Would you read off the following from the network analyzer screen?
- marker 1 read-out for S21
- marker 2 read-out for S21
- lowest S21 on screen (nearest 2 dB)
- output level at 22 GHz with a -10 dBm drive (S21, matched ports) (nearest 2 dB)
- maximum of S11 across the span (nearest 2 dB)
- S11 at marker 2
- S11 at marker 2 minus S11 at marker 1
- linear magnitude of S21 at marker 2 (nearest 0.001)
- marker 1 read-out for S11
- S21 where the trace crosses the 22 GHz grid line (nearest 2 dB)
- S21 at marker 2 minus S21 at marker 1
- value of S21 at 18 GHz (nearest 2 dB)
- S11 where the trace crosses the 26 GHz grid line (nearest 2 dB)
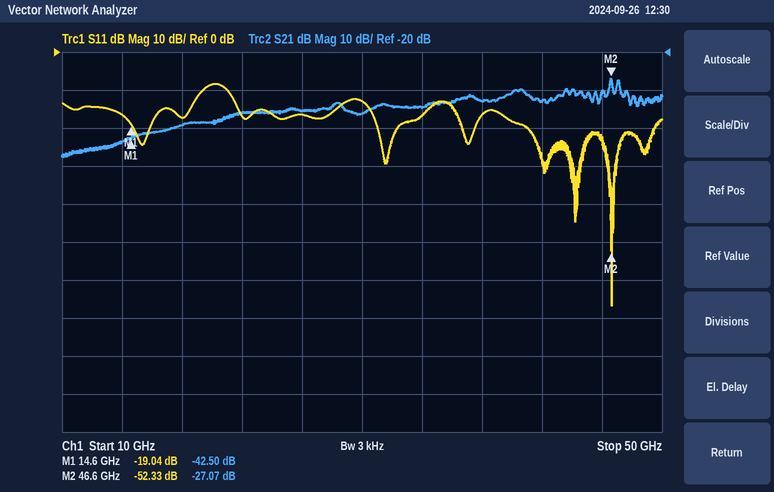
-42.50 dB
-27.07 dB
-48 dB
-46 dBm
-8 dB
-52.33 dB
-33.29 dB
0.044
-19.04 dB
-36 dB
15.43 dB
-40 dB
-16 dB
